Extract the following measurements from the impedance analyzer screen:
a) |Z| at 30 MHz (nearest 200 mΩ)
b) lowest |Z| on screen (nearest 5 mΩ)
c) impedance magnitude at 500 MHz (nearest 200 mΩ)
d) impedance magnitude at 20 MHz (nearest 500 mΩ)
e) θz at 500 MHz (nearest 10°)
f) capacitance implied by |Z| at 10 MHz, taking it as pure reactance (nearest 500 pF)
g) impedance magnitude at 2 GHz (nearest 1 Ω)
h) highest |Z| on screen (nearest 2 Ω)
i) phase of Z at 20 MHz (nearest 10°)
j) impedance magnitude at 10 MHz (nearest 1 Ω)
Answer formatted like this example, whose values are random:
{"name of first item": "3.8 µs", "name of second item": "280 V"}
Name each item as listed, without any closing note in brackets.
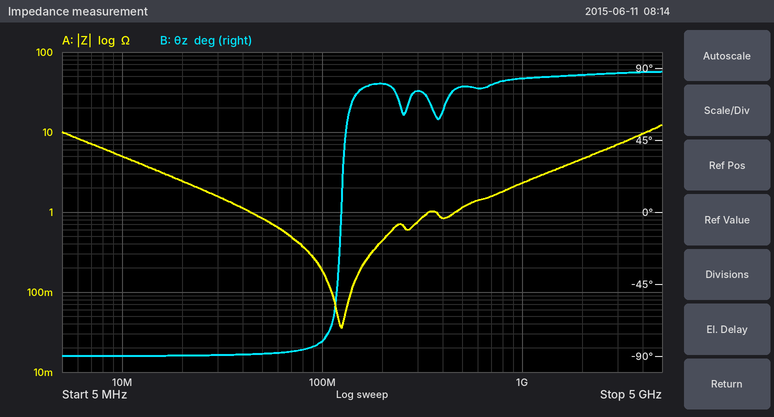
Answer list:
{"|Z| at 30 MHz": "1.6 Ω", "lowest |Z| on screen": "35 mΩ", "impedance magnitude at 500 MHz": "1.2 Ω", "impedance magnitude at 20 MHz": "2.5 Ω", "θz at 500 MHz": "80°", "capacitance implied by |Z| at 10 MHz, taking it as pure reactance": "3.0 nF", "impedance magnitude at 2 GHz": "5 Ω", "highest |Z| on screen": "12 Ω", "phase of Z at 20 MHz": "-90°", "impedance magnitude at 10 MHz": "5 Ω"}
